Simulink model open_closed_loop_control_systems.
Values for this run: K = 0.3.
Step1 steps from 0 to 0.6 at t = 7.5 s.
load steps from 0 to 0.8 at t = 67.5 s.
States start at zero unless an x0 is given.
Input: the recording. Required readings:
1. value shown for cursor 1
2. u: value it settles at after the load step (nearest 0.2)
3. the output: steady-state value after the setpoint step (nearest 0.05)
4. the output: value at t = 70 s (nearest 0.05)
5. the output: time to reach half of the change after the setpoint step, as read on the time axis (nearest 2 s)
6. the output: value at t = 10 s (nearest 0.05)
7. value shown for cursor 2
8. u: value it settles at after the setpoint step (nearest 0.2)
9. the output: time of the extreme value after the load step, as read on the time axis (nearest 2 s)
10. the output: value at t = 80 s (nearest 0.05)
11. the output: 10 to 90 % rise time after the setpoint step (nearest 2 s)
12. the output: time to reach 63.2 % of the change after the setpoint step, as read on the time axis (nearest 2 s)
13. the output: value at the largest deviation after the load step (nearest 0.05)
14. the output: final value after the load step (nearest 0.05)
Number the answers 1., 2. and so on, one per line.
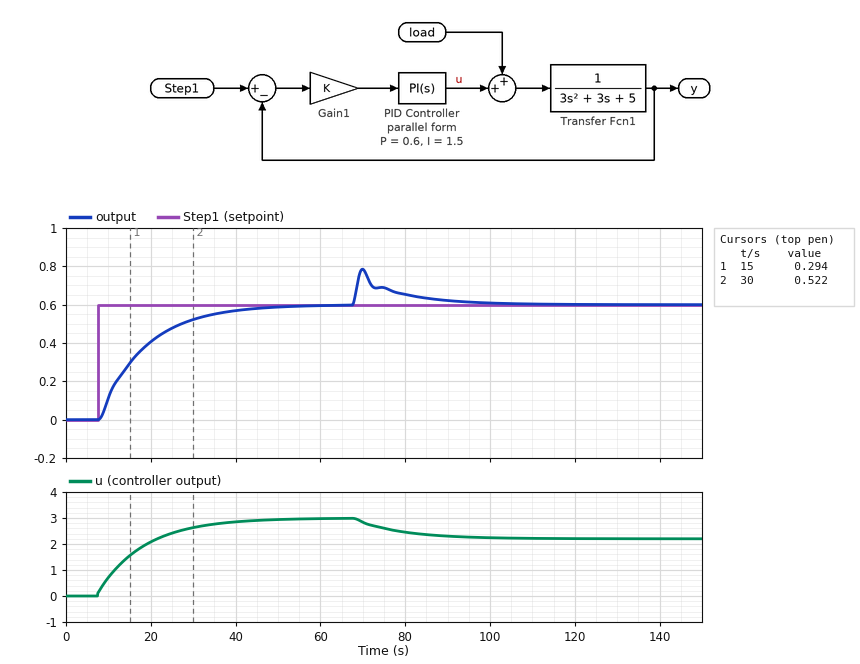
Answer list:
1. 0.294
2. 2.2
3. 0.60
4. 0.80
5. 16 s
6. 0.10
7. 0.522
8. 3.0
9. 70 s
10. 0.65
11. 24 s
12. 18 s
13. 0.80
14. 0.60
